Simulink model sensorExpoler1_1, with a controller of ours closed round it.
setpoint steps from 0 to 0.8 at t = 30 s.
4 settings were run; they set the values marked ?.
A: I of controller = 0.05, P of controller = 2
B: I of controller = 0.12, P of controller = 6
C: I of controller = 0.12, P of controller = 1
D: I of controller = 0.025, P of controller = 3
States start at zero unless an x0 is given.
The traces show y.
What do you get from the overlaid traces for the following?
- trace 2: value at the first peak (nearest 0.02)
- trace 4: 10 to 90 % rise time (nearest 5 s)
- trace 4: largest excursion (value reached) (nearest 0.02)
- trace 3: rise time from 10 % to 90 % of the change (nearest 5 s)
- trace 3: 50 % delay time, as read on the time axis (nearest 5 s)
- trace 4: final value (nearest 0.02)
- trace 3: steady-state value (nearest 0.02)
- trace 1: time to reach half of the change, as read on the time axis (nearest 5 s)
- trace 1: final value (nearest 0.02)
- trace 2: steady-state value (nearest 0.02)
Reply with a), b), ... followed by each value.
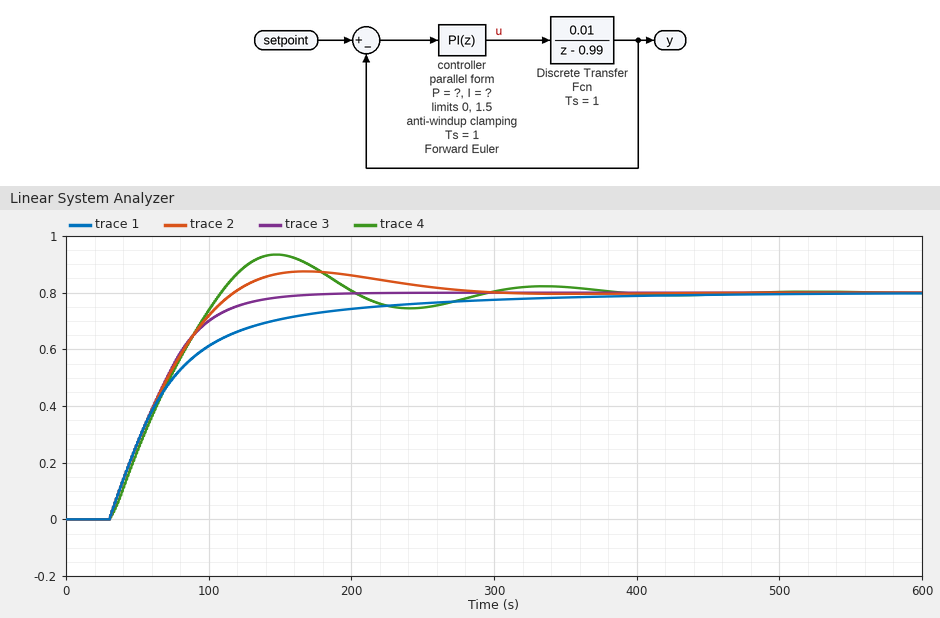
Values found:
a) 0.88
b) 60 s
c) 0.94
d) 70 s
e) 60 s
f) 0.80
g) 0.80
h) 60 s
i) 0.80
j) 0.80
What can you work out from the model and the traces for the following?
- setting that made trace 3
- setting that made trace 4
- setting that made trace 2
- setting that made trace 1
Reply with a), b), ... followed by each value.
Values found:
a) B
b) C
c) A
d) D
